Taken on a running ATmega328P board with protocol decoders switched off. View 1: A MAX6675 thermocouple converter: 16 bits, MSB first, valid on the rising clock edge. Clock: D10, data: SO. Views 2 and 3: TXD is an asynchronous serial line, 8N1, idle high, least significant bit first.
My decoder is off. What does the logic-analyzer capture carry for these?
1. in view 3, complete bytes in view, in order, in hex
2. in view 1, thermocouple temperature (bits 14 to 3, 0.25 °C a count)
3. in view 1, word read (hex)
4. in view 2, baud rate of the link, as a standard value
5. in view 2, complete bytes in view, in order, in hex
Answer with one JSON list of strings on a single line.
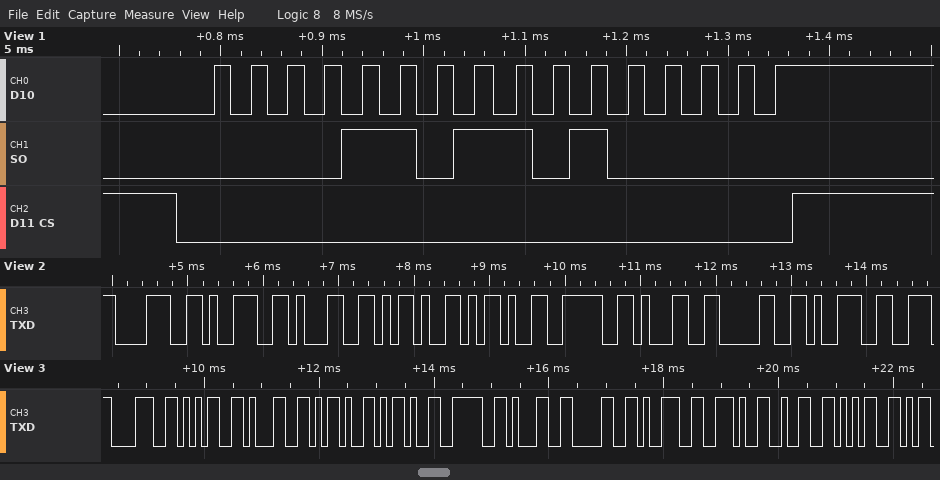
["38 35 31 2D 2D 3E 31 30 39 2E 32 35", "109.00 °C", "0x0DA0", "9600 baud", "0x38 0x39 0x31 0x2D 0x2D 0x3E 0x31 0x30 0x39"]
